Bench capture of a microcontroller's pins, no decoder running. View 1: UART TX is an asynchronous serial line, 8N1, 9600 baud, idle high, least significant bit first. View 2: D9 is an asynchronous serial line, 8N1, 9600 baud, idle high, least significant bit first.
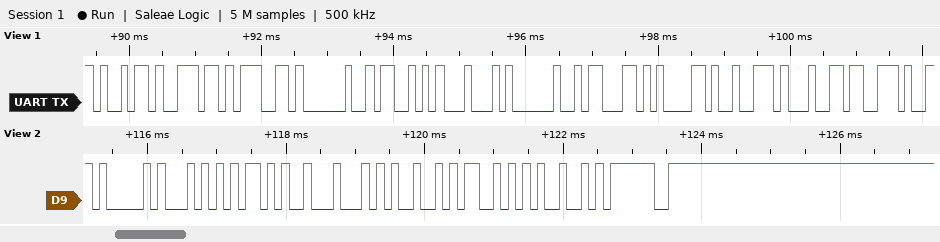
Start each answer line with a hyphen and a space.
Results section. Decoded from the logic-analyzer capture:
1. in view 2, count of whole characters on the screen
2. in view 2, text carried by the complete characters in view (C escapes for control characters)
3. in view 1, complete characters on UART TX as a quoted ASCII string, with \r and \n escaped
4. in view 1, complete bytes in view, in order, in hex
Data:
- 8
- "AT+DISI?"
- "ing SD card."
- 0x69 0x6E 0x67 0x20 0x53 0x44 0x20 0x63 0x61 0x72 0x64 0x2E
